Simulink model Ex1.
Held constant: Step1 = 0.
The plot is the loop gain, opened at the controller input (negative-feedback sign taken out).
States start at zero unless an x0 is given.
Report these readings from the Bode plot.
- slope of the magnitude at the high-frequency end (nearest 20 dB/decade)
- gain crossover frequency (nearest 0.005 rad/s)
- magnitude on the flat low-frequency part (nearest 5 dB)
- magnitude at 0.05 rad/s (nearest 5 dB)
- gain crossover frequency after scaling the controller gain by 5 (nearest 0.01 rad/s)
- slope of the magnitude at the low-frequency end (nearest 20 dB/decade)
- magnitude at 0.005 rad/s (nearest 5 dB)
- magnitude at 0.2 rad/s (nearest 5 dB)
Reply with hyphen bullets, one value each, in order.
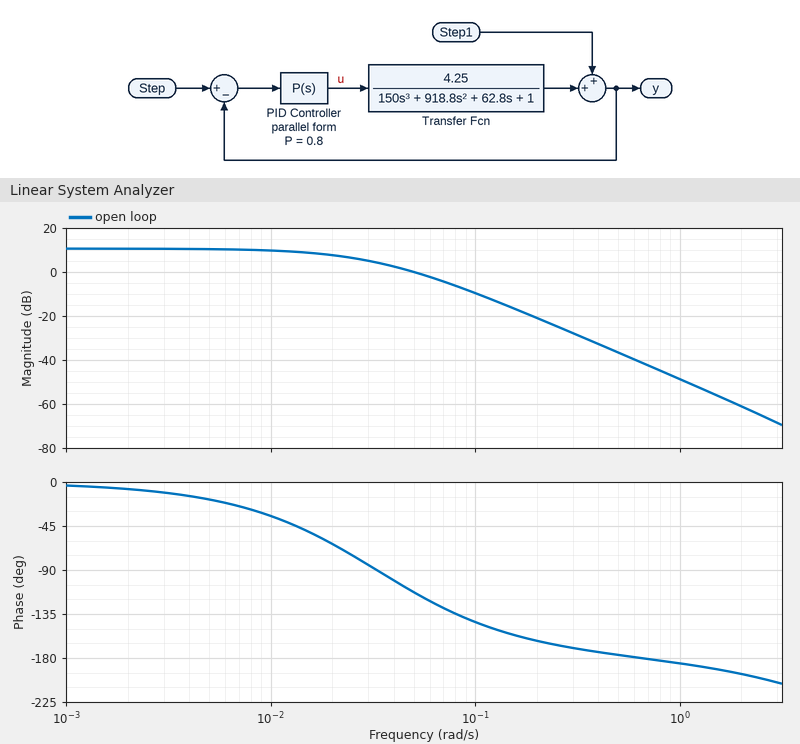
- -40 dB/decade
- 0.050 rad/s
- 10 dB
- 0 dB
- 0.13 rad/s
- 0 dB/decade
- 10 dB
- -20 dB
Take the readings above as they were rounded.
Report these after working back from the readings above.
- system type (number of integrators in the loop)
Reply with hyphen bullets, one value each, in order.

- 0
